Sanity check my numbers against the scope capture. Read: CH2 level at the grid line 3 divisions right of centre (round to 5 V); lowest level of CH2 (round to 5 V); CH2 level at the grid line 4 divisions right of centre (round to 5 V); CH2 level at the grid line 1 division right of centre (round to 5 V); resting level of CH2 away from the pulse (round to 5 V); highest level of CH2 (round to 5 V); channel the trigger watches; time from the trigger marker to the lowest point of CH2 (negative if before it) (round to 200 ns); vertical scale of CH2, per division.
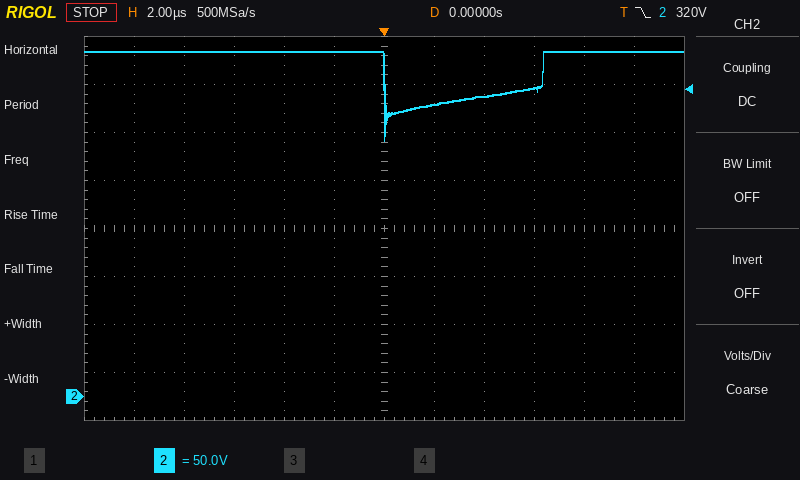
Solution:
320 V
265 V
360 V
305 V
360 V
360 V
CH2
0.0 µs
50 V
